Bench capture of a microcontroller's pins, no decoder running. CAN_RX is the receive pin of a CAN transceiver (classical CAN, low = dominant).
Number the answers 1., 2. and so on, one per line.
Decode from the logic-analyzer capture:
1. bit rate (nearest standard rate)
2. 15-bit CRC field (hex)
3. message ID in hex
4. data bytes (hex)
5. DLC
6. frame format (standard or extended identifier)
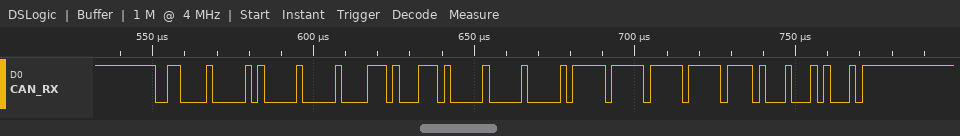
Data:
1. 500 kbit/s
2. 0x2228
3. 0x308
4. 00 1D 1D 00 00 FF FF FF
5. 8
6. standard
